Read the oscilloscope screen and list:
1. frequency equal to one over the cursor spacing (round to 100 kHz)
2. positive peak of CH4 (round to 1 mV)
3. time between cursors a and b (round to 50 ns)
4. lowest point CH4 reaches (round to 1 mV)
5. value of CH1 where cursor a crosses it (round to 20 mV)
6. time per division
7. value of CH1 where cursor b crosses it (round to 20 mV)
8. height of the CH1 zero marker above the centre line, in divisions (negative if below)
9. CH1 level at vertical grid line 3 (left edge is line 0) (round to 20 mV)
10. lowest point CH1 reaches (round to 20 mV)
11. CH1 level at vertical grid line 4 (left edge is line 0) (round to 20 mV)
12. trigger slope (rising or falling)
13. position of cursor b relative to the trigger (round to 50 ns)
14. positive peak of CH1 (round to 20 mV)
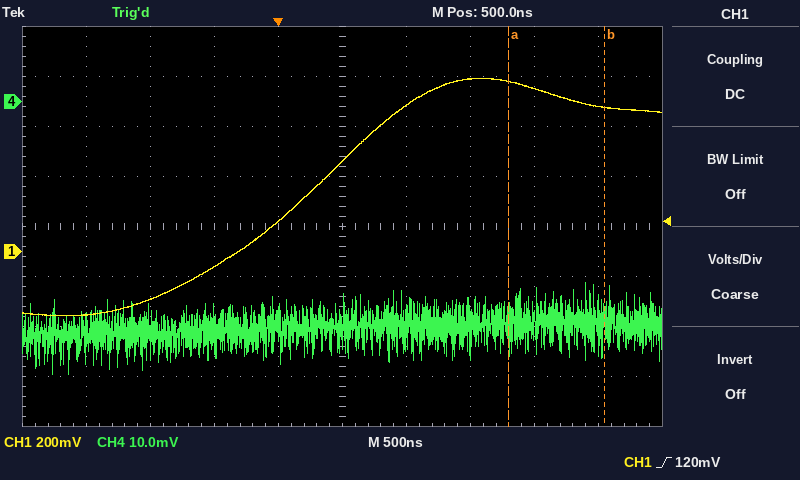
1.3 MHz
-36 mV
750 ns
-55 mV
680 mV
500 ns
580 mV
-0.5 div
-60 mV
-260 mV
120 mV
rising
+2.55 µs
700 mV
